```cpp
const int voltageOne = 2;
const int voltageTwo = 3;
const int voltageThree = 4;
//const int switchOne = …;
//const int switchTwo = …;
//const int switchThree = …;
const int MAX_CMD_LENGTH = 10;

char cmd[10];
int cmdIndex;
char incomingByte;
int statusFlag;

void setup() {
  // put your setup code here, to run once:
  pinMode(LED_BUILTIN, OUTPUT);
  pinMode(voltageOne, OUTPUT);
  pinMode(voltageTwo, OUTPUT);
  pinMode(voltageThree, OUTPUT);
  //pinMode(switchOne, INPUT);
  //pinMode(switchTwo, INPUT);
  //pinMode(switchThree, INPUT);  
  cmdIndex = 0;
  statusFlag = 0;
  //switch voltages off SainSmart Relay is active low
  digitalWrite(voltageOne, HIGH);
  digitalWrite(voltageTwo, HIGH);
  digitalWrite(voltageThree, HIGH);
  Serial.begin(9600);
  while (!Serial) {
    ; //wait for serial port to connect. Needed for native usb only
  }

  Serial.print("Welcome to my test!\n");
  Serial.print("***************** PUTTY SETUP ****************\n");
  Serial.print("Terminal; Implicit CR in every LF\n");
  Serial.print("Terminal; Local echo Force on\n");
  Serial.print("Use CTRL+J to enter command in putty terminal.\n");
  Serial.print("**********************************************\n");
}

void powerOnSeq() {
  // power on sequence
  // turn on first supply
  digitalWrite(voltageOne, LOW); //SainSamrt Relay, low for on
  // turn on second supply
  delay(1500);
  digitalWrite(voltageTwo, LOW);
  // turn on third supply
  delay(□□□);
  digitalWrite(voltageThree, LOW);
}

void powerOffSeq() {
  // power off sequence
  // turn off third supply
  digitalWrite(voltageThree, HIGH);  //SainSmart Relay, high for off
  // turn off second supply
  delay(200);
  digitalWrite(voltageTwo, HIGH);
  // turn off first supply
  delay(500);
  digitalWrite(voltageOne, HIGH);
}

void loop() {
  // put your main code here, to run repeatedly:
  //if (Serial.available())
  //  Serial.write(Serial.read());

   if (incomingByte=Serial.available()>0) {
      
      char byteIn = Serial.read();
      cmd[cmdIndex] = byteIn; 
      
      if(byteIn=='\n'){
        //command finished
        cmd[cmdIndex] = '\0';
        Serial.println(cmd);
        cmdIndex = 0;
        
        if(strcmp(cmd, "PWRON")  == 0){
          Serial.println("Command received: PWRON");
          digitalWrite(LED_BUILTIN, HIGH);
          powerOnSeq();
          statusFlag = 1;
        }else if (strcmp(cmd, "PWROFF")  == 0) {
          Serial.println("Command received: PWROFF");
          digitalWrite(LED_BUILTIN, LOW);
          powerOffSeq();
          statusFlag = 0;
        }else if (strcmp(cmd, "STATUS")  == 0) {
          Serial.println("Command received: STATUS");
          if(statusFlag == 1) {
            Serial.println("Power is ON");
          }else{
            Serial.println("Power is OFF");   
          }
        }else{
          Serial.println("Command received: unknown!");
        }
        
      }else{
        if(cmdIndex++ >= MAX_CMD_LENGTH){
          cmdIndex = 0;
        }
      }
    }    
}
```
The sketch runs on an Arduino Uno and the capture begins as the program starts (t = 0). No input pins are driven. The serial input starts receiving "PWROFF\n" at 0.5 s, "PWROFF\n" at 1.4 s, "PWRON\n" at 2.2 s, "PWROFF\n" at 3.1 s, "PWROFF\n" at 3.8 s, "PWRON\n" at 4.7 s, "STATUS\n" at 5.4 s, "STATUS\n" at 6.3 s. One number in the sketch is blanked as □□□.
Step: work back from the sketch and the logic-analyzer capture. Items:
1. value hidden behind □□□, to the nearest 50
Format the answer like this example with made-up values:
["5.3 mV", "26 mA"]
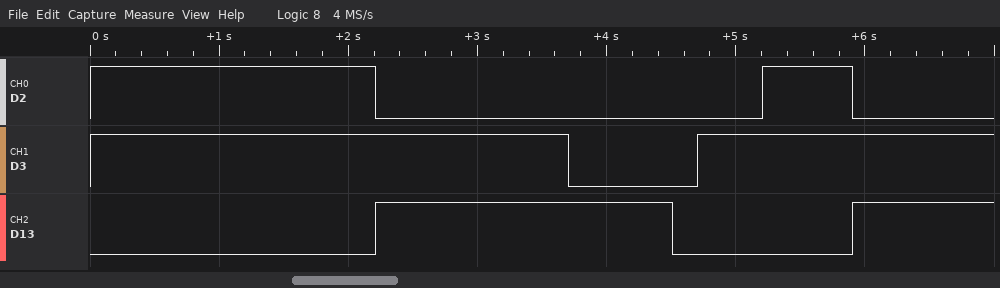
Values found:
["800"]
